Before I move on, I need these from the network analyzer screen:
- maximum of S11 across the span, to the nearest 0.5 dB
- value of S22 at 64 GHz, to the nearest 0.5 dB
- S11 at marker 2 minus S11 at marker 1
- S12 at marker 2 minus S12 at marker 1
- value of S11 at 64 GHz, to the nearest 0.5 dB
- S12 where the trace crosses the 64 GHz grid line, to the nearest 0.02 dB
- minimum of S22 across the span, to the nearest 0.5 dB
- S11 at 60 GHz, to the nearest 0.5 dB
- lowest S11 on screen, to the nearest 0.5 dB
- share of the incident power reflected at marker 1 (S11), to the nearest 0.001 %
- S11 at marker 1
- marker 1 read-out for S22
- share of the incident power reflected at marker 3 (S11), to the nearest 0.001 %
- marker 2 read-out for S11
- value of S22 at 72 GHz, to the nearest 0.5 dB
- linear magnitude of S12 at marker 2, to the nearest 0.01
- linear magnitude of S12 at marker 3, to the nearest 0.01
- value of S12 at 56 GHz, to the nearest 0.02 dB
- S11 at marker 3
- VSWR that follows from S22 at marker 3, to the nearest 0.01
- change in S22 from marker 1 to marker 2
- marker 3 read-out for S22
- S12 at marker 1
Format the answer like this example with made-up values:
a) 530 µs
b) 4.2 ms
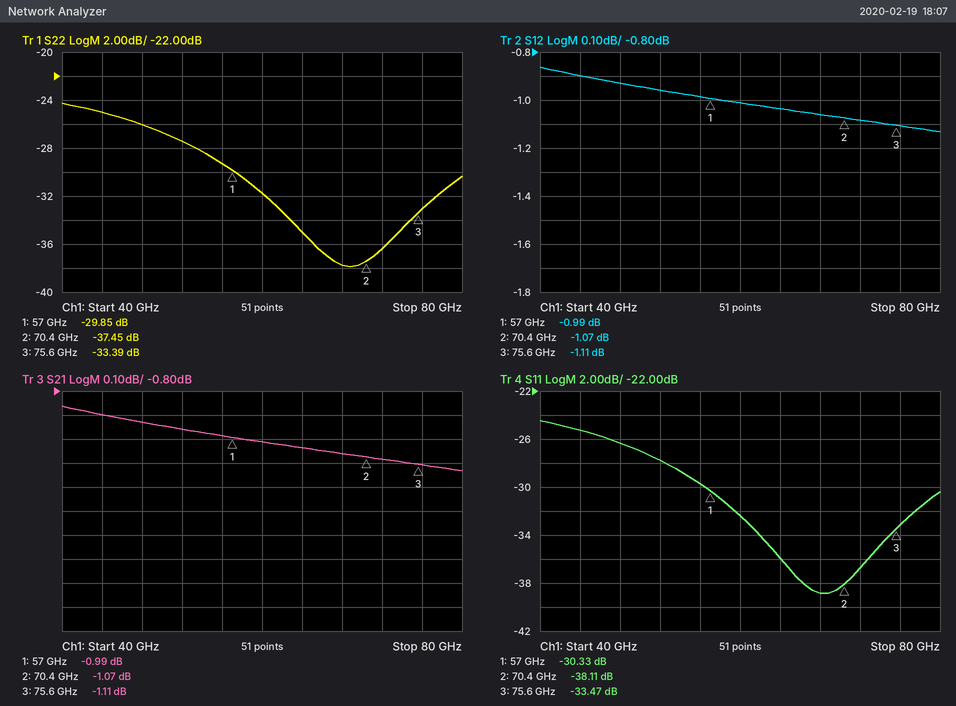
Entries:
a) -24.5 dB
b) -35.0 dB
c) -7.78 dB
d) -0.08 dB
e) -36.0 dB
f) -1.04 dB
g) -38.0 dB
h) -32.5 dB
i) -39.0 dB
j) 0.093 %
k) -30.33 dB
l) -29.85 dB
m) 0.045 %
n) -38.11 dB
o) -36.5 dB
p) 0.88
q) 0.88
r) -0.98 dB
s) -33.47 dB
t) 1.04
u) -7.60 dB
v) -33.39 dB
w) -0.99 dB
